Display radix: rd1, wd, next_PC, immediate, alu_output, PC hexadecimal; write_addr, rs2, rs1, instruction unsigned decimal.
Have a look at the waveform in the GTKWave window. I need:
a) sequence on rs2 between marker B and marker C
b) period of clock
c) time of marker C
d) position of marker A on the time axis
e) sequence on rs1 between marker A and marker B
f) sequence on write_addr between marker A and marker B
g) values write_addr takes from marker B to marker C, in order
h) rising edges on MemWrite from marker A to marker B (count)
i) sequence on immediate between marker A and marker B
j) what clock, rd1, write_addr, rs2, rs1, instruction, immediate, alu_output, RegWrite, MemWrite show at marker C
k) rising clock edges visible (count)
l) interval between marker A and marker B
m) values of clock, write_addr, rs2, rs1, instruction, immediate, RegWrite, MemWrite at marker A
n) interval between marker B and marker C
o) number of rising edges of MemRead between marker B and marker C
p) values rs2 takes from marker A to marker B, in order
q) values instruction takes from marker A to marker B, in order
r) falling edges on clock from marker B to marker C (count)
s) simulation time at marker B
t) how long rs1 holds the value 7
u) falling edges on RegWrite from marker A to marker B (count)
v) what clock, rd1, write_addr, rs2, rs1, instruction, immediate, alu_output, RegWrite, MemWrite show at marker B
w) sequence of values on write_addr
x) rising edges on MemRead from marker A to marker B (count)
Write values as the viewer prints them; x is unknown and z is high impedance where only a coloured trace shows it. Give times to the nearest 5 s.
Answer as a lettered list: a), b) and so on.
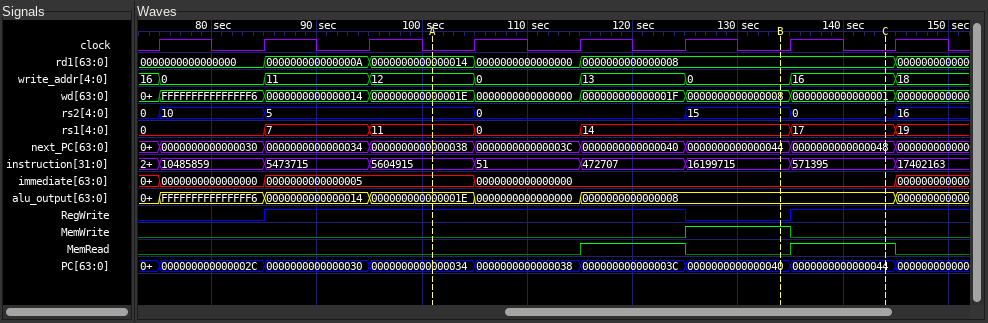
a) 15, 0
b) 10 s
c) 145 s
d) 100 s
e) 11, 0, 14
f) 12, 0, 13, 0
g) 0, 16
h) 1
i) 0000000000000005, 0000000000000000
j) clock=0, rd1=0000000000000008, write_addr=16, rs2=0, rs1=17, instruction=571395, immediate=0000000000000000, alu_output=0000000000000008, RegWrite=1, MemWrite=0
k) 8
l) 35 s
m) clock=0, write_addr=12, rs2=5, rs1=11, instruction=5604915, immediate=0000000000000005, RegWrite=1, MemWrite=0
n) 10 s
o) 1
p) 5, 0, 15
q) 5604915, 51, 472707, 16199715
r) 1
s) 135 s
t) 10 s
u) 1
v) clock=0, rd1=0000000000000008, write_addr=0, rs2=15, rs1=14, instruction=16199715, immediate=0000000000000000, alu_output=0000000000000008, RegWrite=0, MemWrite=1
w) 16, 0, 11, 12, 0, 13, 0, 16, 18
x) 1
